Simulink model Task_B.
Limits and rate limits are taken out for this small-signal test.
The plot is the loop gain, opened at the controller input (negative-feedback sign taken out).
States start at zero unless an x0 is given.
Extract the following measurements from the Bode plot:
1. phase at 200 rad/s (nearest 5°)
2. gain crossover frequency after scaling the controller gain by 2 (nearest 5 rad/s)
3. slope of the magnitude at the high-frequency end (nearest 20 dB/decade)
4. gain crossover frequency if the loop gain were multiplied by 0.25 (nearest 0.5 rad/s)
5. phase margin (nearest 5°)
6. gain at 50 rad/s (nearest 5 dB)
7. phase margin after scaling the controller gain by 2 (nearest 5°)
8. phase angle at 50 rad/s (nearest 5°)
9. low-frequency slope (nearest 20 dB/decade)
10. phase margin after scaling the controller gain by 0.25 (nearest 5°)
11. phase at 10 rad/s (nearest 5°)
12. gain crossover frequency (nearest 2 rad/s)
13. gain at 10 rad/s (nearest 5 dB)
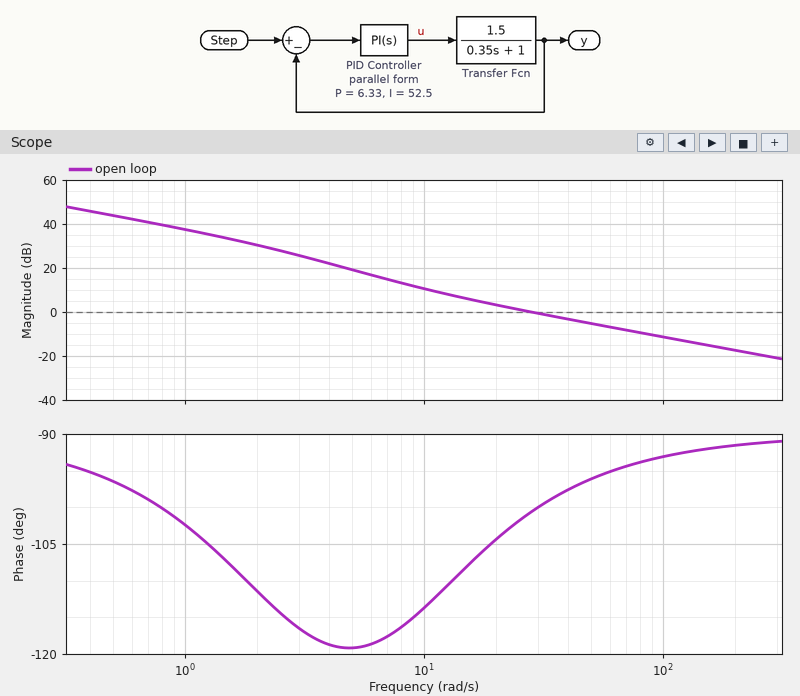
-90°
55 rad/s
-20 dB/decade
9.0 rad/s
80°
-5 dB
85°
-95°
-20 dB/decade
65°
-115°
28 rad/s
10 dB
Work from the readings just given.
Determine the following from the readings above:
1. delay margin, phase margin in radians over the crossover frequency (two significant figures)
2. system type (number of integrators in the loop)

0.050 s
1
